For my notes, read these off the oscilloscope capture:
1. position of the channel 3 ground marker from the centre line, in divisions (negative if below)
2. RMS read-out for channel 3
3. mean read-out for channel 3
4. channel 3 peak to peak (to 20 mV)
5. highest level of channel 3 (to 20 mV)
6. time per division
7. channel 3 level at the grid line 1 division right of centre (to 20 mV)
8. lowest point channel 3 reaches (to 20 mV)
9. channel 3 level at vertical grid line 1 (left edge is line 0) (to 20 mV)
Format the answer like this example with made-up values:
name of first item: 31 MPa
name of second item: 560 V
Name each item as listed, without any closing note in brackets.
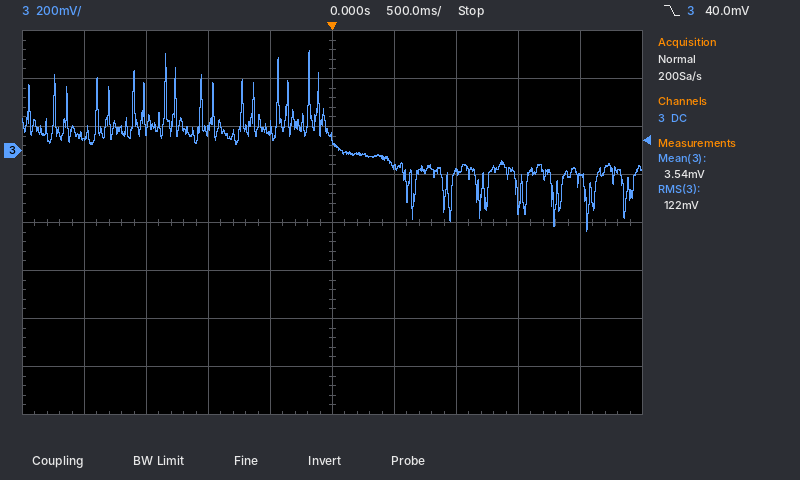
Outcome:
position of the channel 3 ground marker from the centre line, in divisions: +1.5 div
RMS read-out for channel 3: 122 mV
mean read-out for channel 3: 3.54 mV
channel 3 peak to peak: 760 mV
highest level of channel 3: 420 mV
time per division: 500 ms
channel 3 level at the grid line 1 division right of centre: -60 mV
lowest point channel 3 reaches: -340 mV
channel 3 level at vertical grid line 1 (left edge is line 0): 60 mV
